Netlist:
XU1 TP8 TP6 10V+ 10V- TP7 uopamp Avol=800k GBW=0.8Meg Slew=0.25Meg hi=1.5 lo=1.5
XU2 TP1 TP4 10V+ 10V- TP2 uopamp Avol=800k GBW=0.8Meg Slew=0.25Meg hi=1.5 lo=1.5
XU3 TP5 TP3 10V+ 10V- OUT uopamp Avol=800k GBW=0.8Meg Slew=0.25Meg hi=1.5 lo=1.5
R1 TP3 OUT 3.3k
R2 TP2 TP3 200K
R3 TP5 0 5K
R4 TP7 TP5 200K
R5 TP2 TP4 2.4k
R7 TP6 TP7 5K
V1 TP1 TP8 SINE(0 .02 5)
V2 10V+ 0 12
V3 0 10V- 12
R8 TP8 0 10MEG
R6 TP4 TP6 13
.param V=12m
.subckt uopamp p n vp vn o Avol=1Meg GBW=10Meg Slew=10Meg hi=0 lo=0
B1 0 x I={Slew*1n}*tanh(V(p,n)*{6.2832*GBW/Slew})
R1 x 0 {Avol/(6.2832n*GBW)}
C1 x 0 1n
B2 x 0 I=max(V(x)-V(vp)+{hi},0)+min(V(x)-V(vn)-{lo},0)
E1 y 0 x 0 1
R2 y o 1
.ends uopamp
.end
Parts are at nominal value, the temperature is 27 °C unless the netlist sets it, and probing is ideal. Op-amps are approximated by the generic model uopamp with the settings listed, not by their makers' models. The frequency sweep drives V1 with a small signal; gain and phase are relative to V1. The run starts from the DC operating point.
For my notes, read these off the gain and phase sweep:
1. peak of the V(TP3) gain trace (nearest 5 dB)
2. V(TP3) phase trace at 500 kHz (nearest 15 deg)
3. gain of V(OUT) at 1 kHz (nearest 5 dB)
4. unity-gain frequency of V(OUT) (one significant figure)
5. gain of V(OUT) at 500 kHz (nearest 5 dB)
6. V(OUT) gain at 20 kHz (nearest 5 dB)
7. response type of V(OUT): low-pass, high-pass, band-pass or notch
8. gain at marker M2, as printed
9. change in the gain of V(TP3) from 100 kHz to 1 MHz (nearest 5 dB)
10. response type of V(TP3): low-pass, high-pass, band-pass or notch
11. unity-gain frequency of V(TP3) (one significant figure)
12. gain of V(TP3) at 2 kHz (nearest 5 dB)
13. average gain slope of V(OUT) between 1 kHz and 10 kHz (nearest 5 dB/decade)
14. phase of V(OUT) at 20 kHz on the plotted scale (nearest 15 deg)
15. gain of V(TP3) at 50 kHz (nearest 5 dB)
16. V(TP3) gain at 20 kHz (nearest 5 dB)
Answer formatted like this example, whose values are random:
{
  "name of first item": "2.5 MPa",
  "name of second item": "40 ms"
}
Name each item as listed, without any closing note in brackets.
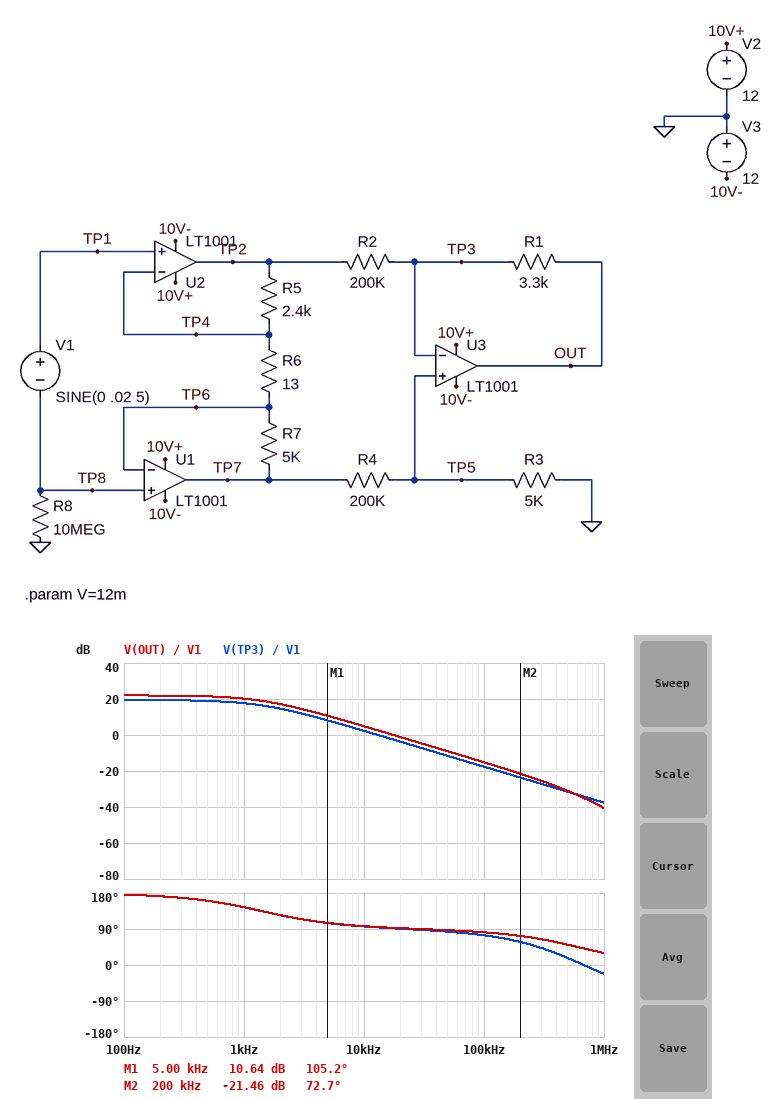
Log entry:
{
  "peak of the V(TP3) gain trace": "20 dB",
  "V(TP3) phase trace at 500 kHz": "15 deg",
  "gain of V(OUT) at 1 kHz": "20 dB",
  "unity-gain frequency of V(OUT)": "20 kHz",
  "gain of V(OUT) at 500 kHz": "-30 dB",
  "V(OUT) gain at 20 kHz": "0 dB",
  "response type of V(OUT): low-pass, high-pass, band-pass or notch": "low-pass",
  "gain at marker M2, as printed": "-21.46 dB",
  "change in the gain of V(TP3) from 100 kHz to 1 MHz": "-20 dB",
  "response type of V(TP3): low-pass, high-pass, band-pass or notch": "low-pass",
  "unity-gain frequency of V(TP3)": "10 kHz",
  "gain of V(TP3) at 2 kHz": "15 dB",
  "average gain slope of V(OUT) between 1 kHz and 10 kHz": "-15 dB/decade",
  "phase of V(OUT) at 20 kHz on the plotted scale": "90 deg",
  "gain of V(TP3) at 50 kHz": "-10 dB",
  "V(TP3) gain at 20 kHz": "-5 dB"
}
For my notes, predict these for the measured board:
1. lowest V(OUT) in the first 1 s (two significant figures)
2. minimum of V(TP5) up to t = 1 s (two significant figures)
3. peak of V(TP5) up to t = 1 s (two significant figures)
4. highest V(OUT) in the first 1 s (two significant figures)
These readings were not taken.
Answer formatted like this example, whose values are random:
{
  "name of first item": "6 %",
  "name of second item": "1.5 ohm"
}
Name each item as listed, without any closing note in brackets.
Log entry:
{
  "lowest V(OUT) in the first 1 s": "-250 mV",
  "minimum of V(TP5) up to t = 1 s": "-190 mV",
  "peak of V(TP5) up to t = 1 s": "190 mV",
  "highest V(OUT) in the first 1 s": "250 mV"
}
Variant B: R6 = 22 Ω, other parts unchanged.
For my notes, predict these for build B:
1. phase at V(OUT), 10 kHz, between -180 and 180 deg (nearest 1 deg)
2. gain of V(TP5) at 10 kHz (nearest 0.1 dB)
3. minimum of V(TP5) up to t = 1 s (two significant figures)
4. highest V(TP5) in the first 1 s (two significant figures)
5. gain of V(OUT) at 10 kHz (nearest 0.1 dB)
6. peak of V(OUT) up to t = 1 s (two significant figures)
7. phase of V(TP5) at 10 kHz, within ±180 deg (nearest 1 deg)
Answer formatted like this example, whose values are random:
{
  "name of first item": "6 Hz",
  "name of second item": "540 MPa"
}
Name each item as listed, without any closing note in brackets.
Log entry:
{
  "phase at V(OUT), 10 kHz, between -180 and 180 deg": "102 deg",
  "gain of V(TP5) at 10 kHz": "2.1 dB",
  "minimum of V(TP5) up to t = 1 s": "-110 mV",
  "highest V(TP5) in the first 1 s": "110 mV",
  "gain of V(OUT) at 10 kHz": "4.7 dB",
  "peak of V(OUT) up to t = 1 s": "150 mV",
  "phase of V(TP5) at 10 kHz, within ±180 deg": "103 deg"
}
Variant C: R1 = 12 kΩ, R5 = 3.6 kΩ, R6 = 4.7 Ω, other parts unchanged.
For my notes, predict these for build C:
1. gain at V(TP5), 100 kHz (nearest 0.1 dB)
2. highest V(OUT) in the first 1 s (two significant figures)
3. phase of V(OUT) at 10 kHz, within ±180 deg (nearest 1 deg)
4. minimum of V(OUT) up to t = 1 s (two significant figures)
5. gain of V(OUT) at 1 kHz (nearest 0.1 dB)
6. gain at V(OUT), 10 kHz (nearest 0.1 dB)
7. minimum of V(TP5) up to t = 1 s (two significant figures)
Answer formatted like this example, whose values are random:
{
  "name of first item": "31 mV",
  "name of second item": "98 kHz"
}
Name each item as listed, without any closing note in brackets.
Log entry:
{
  "gain at V(TP5), 100 kHz": "-19.0 dB",
  "highest V(OUT) in the first 1 s": "730 mV",
  "phase of V(OUT) at 10 kHz, within ±180 deg": "92 deg",
  "minimum of V(OUT) up to t = 1 s": "-730 mV",
  "gain of V(OUT) at 1 kHz": "29.4 dB",
  "gain at V(OUT), 10 kHz": "10.1 dB",
  "minimum of V(TP5) up to t = 1 s": "-260 mV"
}
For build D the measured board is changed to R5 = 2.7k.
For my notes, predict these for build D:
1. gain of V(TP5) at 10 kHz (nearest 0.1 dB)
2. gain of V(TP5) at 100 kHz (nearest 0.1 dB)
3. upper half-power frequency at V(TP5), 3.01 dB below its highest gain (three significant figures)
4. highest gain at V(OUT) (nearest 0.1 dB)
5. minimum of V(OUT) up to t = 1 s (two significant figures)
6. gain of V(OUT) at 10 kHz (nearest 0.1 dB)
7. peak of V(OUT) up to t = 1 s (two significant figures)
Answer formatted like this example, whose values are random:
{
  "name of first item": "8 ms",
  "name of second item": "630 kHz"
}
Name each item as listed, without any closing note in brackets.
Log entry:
{
  "gain of V(TP5) at 10 kHz": "2.0 dB",
  "gain of V(TP5) at 100 kHz": "-18.0 dB",
  "upper half-power frequency at V(TP5), 3.01 dB below its highest gain": "1.35 kHz",
  "highest gain at V(OUT)": "22.3 dB",
  "minimum of V(OUT) up to t = 1 s": "-260 mV",
  "gain of V(OUT) at 10 kHz": "4.8 dB",
  "peak of V(OUT) up to t = 1 s": "260 mV"
}
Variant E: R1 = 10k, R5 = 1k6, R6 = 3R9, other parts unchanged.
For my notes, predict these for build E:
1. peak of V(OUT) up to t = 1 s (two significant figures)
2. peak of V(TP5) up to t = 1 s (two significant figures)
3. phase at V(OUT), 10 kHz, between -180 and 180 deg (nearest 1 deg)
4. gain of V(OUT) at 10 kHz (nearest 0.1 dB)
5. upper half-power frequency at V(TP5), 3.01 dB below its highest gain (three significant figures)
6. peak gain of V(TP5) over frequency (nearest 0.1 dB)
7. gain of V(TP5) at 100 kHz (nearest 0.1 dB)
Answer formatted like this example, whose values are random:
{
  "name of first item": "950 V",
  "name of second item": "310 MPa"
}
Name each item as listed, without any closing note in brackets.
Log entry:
{
  "peak of V(OUT) up to t = 1 s": "440 mV",
  "peak of V(TP5) up to t = 1 s": "260 mV",
  "phase at V(OUT), 10 kHz, between -180 and 180 deg": "92 deg",
  "gain of V(OUT) at 10 kHz": "8.0 dB",
  "upper half-power frequency at V(TP5), 3.01 dB below its highest gain": "473 Hz",
  "peak gain of V(TP5) over frequency": "29.9 dB",
  "gain of V(TP5) at 100 kHz": "-16.7 dB"
}
